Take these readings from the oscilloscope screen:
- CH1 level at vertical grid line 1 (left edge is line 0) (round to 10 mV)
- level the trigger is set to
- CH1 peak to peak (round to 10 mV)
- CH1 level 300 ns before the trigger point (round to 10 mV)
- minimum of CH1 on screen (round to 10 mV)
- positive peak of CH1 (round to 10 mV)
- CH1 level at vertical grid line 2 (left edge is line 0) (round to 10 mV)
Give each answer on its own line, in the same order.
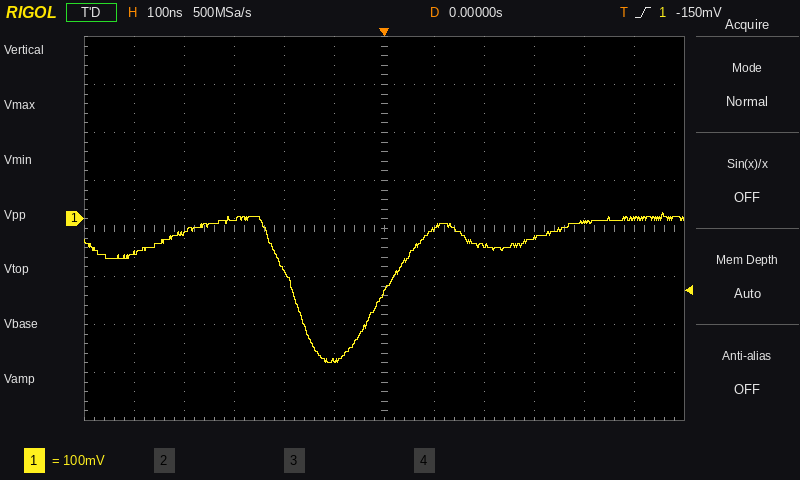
-70 mV
-150 mV
310 mV
0 mV
-300 mV
10 mV
-30 mV
